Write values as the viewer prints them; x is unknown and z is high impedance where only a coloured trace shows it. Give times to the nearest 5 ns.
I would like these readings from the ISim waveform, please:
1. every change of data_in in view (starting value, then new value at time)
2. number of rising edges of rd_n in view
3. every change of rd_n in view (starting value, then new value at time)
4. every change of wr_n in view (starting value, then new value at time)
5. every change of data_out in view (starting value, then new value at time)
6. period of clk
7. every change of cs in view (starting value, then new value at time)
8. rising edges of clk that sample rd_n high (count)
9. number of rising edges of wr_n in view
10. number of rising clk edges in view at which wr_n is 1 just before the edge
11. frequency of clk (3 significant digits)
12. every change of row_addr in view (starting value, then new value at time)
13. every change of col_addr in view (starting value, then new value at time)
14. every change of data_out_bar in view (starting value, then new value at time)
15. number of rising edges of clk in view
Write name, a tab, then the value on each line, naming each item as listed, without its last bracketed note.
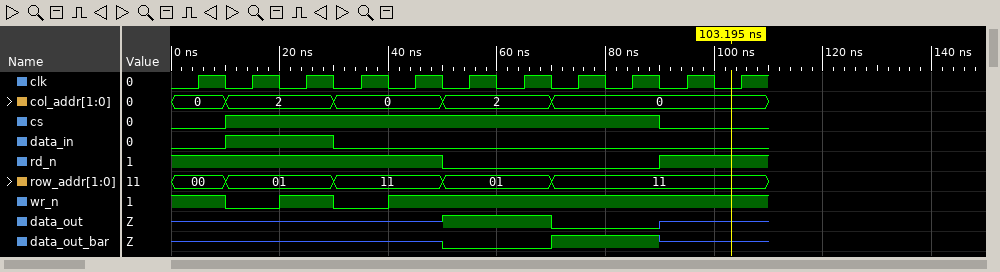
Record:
every change of data_in in view	0, 1 at 10 ns, 0 at 30 ns
number of rising edges of rd_n in view	1
every change of rd_n in view	1, 0 at 50 ns, 1 at 90 ns
every change of wr_n in view	1, 0 at 10 ns, 1 at 20 ns, 0 at 30 ns, 1 at 40 ns
every change of data_out in view	z, 1 at 50 ns, 0 at 70 ns, z at 90 ns
period of clk	10 ns
every change of cs in view	0, 1 at 10 ns, 0 at 90 ns
rising edges of clk that sample rd_n high	7
number of rising edges of wr_n in view	2
number of rising clk edges in view at which wr_n is 1 just before the edge	9
frequency of clk	100 MHz
every change of row_addr in view	00, 01 at 10 ns, 11 at 30 ns, 01 at 50 ns, 11 at 70 ns
every change of col_addr in view	0, 2 at 10 ns, 0 at 30 ns, 2 at 50 ns, 0 at 70 ns
every change of data_out_bar in view	z, 0 at 50 ns, 1 at 70 ns, z at 90 ns
number of rising edges of clk in view	11
